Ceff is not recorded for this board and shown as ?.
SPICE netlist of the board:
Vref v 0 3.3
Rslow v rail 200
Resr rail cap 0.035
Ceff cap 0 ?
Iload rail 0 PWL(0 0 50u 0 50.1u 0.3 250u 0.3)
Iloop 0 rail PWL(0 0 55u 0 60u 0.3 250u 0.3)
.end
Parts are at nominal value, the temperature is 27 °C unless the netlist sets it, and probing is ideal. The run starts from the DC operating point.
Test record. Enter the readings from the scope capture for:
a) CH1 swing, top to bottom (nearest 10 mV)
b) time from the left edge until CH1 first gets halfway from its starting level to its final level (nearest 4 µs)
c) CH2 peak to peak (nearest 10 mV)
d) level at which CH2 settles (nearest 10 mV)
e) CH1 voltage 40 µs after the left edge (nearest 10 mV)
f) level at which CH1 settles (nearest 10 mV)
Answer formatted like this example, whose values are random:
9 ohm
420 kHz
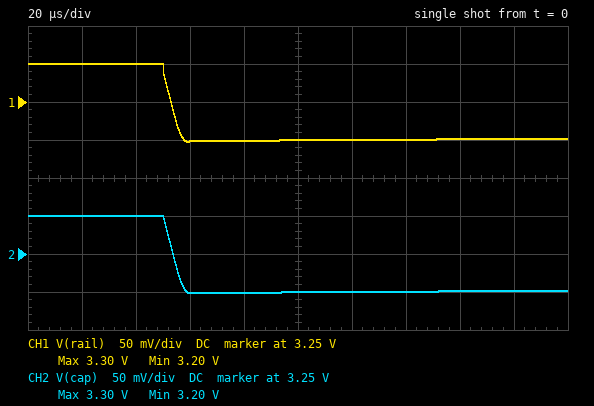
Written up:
100 mV
52 µs
100 mV
3.20 V
3.30 V
3.20 V
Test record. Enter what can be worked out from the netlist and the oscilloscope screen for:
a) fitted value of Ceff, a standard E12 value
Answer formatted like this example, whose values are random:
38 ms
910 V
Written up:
22 µF
